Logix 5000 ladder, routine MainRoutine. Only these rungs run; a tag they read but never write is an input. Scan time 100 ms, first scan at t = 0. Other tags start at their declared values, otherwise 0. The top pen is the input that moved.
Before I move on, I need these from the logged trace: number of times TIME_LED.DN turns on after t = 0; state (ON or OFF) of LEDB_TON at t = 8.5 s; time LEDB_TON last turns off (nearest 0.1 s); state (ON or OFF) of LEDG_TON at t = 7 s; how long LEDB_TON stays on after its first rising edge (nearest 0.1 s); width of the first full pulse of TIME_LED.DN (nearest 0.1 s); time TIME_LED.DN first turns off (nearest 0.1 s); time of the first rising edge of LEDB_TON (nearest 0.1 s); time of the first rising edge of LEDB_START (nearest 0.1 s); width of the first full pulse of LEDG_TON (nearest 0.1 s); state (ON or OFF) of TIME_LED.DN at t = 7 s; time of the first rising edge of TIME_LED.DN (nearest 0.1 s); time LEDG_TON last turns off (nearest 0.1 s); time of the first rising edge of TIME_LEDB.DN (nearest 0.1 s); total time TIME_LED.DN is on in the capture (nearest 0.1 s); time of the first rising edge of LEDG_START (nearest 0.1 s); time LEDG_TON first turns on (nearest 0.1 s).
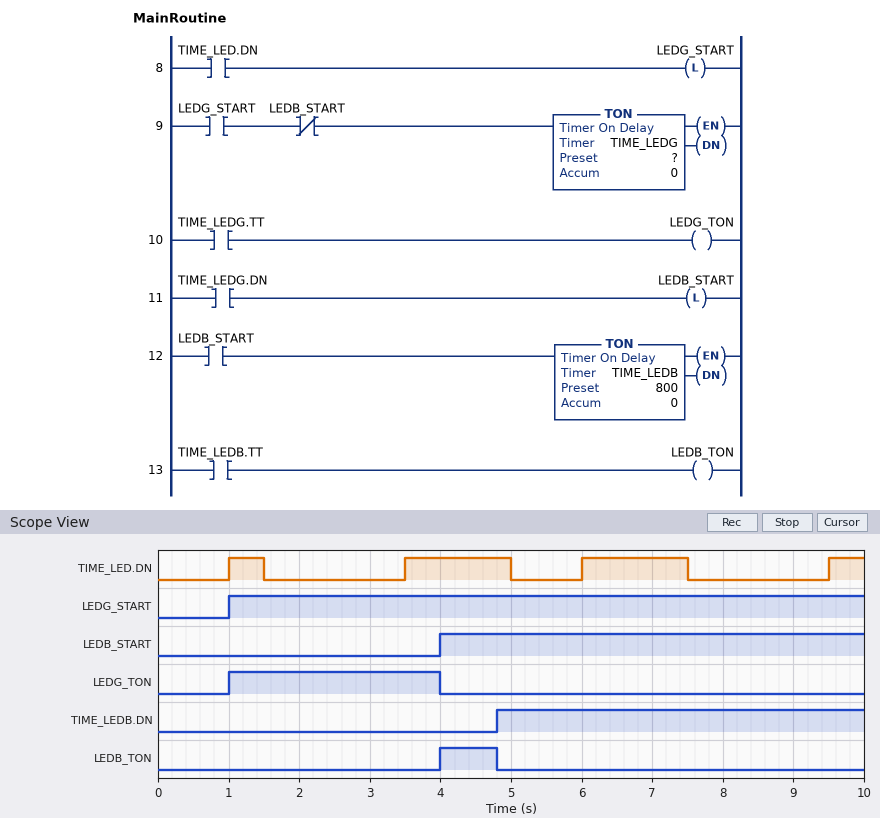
4
OFF
4.8 s
OFF
0.8 s
0.5 s
1.5 s
4.0 s
4.0 s
3.0 s
ON
1.0 s
4.0 s
4.8 s
4.0 s
1.0 s
1.0 s
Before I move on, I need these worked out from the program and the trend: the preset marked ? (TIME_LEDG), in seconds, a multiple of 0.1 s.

3.0 s
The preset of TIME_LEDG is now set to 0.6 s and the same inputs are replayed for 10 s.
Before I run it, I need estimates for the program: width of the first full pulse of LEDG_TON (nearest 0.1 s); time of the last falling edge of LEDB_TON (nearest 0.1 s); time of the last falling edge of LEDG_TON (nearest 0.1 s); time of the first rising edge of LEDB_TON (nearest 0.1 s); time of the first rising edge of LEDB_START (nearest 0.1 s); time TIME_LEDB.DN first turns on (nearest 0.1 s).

0.6 s
2.4 s
1.6 s
1.6 s
1.6 s
2.4 s
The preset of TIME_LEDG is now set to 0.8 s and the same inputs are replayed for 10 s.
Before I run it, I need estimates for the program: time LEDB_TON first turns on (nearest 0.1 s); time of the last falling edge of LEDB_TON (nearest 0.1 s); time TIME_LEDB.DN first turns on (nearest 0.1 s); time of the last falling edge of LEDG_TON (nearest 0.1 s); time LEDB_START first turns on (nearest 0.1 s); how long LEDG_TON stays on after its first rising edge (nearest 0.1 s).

1.8 s
2.6 s
2.6 s
1.8 s
1.8 s
0.8 s
